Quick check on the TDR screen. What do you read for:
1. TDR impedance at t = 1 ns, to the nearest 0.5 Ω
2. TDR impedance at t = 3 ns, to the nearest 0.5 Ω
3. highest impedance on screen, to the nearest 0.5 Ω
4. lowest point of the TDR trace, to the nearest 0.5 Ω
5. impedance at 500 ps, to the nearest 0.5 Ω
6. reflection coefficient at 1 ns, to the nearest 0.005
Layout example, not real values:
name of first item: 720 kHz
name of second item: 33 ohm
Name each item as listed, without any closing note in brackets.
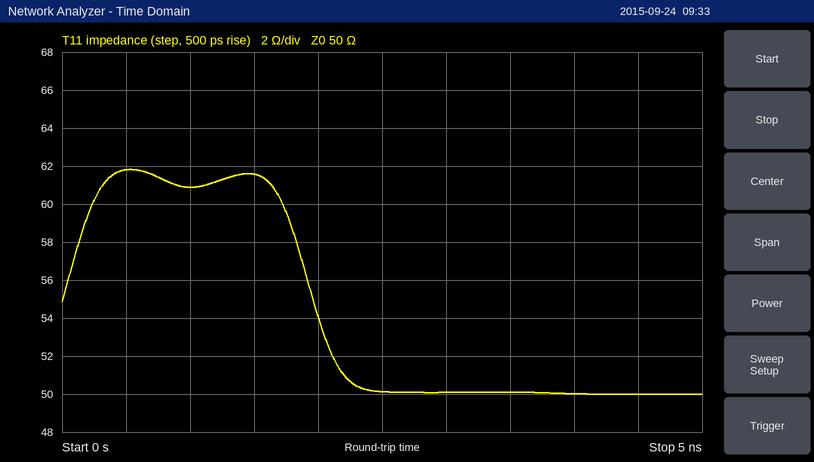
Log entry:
TDR impedance at t = 1 ns, to the nearest 0.5 Ω: 61.0 Ω
TDR impedance at t = 3 ns, to the nearest 0.5 Ω: 50.0 Ω
highest impedance on screen, to the nearest 0.5 Ω: 62.0 Ω
lowest point of the TDR trace, to the nearest 0.5 Ω: 50.0 Ω
impedance at 500 ps, to the nearest 0.5 Ω: 62.0 Ω
reflection coefficient at 1 ns, to the nearest 0.005: +0.100
